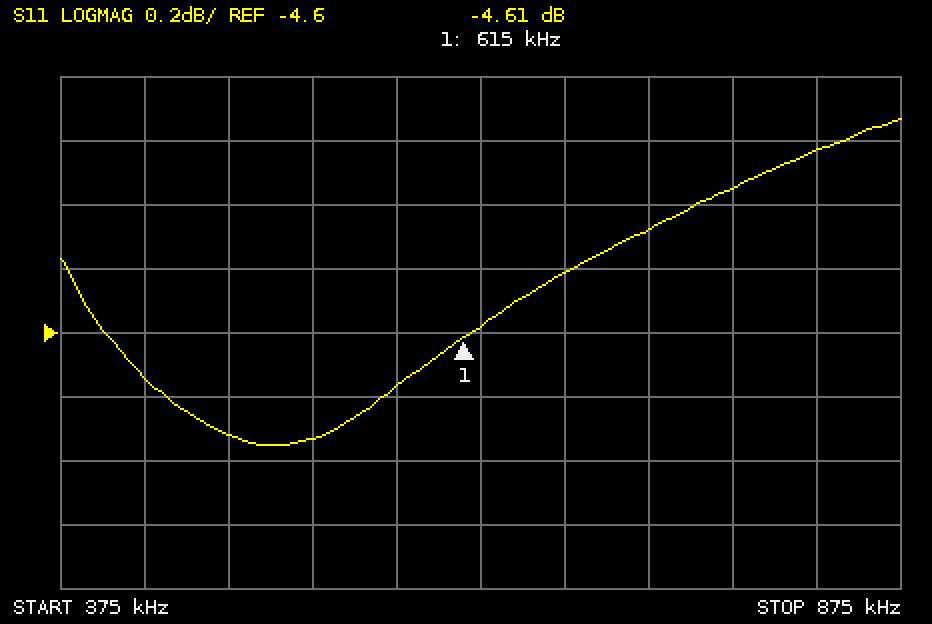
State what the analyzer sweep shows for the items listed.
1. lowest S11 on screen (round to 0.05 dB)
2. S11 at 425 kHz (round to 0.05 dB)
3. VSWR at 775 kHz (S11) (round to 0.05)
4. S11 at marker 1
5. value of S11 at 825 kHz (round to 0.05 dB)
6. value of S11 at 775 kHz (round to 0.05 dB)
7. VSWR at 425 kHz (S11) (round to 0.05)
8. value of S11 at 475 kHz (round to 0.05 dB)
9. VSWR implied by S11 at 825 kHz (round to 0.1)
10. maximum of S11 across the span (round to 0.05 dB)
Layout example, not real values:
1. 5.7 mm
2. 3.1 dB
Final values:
1. -4.95 dB
2. -4.75 dB
3. 4.25
4. -4.61 dB
5. -4.05 dB
6. -4.15 dB
7. 3.75
8. -4.90 dB
9. 4.4
10. -3.95 dB
